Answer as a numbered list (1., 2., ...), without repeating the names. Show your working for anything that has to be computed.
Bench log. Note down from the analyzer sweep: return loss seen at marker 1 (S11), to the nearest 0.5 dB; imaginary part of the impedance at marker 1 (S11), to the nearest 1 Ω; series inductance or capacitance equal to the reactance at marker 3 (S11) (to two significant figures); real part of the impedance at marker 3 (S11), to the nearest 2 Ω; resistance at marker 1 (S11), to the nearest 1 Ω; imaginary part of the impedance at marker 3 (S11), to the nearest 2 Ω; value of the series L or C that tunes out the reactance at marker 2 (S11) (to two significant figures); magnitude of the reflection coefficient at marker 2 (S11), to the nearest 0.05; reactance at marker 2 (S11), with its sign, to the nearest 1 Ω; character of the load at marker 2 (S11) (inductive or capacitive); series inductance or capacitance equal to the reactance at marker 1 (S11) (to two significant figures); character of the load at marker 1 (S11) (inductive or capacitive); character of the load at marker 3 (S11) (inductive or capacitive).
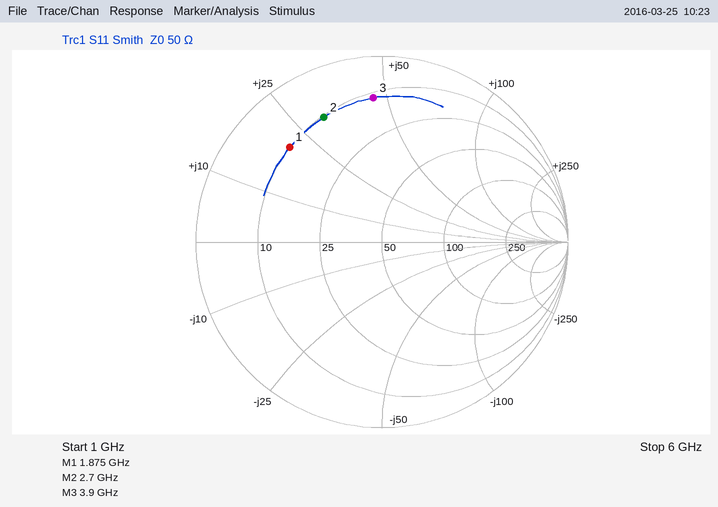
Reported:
1. 3.0 dB
2. +20 Ω
3. L = 46 Ω/(2π × 3.9 GHz) ≈ 1.9 nH
4. 12 Ω
5. 10 Ω
6. +46 Ω
7. C = 1/(2π × 2.7 GHz × 31 Ω) ≈ 1.9 pF
8. 0.75
9. +31 Ω
10. inductive
11. L = 20 Ω/(2π × 1.875 GHz) ≈ 1.7 nH
12. inductive
13. inductive
